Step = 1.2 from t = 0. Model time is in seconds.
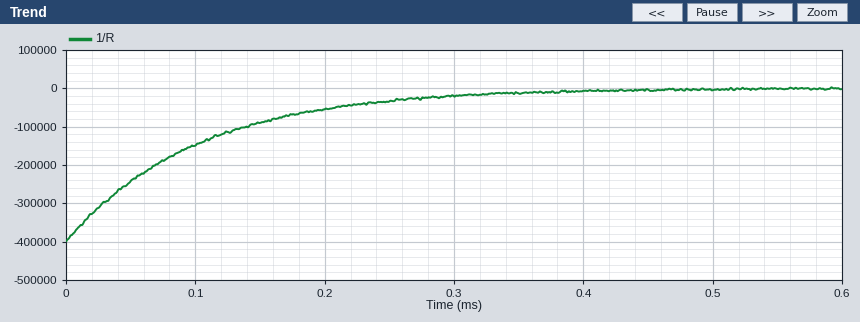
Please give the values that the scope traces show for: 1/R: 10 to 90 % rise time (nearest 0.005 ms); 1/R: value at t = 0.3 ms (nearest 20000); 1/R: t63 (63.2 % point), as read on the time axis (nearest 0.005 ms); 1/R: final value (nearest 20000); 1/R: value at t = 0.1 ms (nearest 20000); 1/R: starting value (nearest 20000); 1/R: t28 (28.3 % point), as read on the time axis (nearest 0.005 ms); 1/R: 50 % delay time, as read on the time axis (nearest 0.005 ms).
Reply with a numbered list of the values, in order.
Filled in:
1. 0.220 ms
2. -20000
3. 0.100 ms
4. 0
5. -140000
6. -400000
7. 0.035 ms
8. 0.070 ms
